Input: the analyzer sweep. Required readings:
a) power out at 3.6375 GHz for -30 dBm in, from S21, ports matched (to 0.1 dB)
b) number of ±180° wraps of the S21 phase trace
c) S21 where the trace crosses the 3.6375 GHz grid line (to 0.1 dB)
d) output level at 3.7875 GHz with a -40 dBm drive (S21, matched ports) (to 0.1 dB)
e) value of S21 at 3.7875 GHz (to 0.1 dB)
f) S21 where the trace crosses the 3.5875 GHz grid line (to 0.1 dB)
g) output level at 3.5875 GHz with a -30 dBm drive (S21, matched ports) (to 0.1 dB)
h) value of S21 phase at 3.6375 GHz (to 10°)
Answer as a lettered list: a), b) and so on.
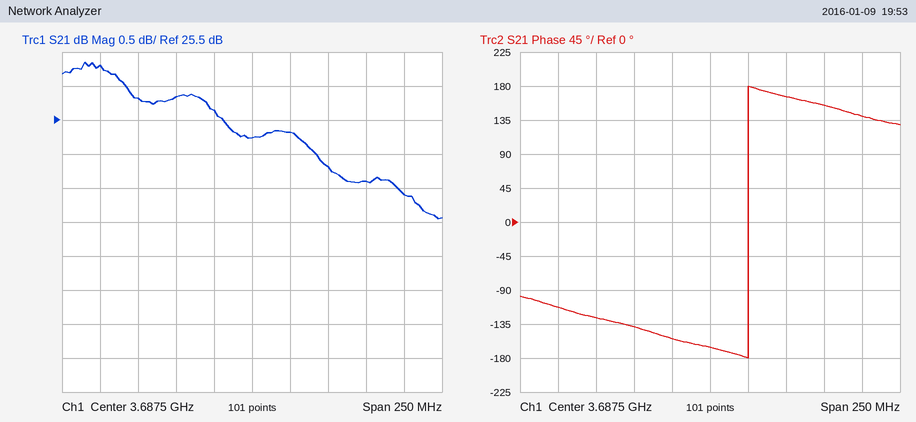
a) -4.2 dBm
b) 1
c) 25.8 dB
d) -15.6 dBm
e) 24.4 dB
f) 26.3 dB
g) -3.7 dBm
h) -140°
